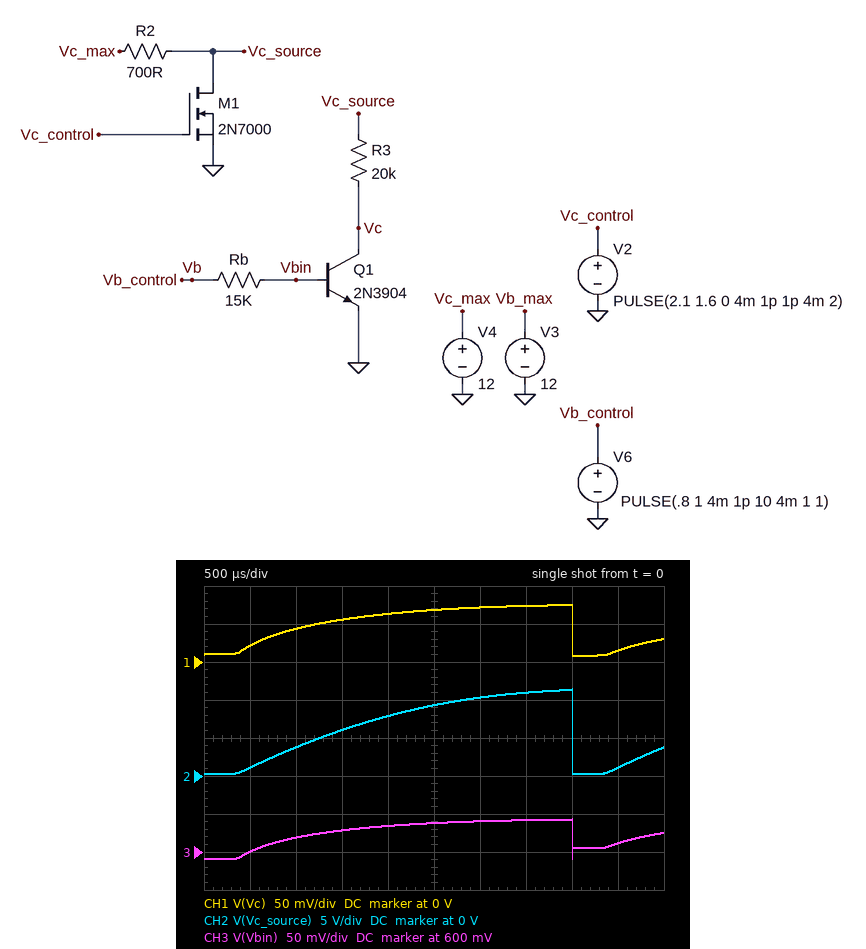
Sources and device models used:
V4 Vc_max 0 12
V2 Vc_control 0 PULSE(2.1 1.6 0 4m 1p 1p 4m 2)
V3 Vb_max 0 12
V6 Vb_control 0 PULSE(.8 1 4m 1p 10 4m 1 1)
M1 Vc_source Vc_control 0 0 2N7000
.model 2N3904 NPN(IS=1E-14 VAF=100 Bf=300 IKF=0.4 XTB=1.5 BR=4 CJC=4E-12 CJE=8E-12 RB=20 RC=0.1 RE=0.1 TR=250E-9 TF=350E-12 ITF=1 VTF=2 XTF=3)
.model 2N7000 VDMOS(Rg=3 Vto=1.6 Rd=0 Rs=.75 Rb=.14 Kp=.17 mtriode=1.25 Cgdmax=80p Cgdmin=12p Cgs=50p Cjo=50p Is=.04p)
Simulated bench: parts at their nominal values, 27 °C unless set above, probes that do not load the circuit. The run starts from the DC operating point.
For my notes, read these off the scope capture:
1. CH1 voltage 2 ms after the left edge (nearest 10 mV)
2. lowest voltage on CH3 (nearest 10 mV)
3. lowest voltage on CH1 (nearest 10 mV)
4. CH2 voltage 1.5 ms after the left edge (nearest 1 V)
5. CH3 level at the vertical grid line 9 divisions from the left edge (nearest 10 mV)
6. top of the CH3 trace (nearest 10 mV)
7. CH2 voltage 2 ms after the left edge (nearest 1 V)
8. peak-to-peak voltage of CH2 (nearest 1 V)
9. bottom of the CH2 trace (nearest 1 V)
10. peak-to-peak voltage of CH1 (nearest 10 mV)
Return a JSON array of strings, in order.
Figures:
["60 mV", "590 mV", "10 mV", "6 V", "610 mV", "640 mV", "8 V", "11 V", "0 V", "70 mV"]
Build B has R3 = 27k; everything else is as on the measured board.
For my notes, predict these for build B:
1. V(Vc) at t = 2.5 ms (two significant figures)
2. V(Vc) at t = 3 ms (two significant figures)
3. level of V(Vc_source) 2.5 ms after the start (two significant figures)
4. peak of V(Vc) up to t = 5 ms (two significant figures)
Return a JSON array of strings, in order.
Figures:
["60 mV", "63 mV", "9.4 V", "66 mV"]
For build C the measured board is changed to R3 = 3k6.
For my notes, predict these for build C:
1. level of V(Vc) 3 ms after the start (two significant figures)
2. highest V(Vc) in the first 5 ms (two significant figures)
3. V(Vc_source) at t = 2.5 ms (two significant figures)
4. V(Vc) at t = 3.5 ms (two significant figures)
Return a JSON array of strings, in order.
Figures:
["320 mV", "1.3 V", "8.1 V", "930 mV"]
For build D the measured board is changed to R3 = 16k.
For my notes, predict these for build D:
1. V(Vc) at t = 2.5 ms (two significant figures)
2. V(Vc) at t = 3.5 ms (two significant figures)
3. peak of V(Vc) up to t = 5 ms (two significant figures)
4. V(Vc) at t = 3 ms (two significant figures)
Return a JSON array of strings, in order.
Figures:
["75 mV", "81 mV", "83 mV", "79 mV"]
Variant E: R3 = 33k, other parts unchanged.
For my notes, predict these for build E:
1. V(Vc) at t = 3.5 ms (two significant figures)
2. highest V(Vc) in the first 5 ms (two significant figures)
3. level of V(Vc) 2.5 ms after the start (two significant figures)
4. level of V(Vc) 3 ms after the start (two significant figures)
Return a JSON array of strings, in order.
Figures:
["59 mV", "60 mV", "54 mV", "57 mV"]
